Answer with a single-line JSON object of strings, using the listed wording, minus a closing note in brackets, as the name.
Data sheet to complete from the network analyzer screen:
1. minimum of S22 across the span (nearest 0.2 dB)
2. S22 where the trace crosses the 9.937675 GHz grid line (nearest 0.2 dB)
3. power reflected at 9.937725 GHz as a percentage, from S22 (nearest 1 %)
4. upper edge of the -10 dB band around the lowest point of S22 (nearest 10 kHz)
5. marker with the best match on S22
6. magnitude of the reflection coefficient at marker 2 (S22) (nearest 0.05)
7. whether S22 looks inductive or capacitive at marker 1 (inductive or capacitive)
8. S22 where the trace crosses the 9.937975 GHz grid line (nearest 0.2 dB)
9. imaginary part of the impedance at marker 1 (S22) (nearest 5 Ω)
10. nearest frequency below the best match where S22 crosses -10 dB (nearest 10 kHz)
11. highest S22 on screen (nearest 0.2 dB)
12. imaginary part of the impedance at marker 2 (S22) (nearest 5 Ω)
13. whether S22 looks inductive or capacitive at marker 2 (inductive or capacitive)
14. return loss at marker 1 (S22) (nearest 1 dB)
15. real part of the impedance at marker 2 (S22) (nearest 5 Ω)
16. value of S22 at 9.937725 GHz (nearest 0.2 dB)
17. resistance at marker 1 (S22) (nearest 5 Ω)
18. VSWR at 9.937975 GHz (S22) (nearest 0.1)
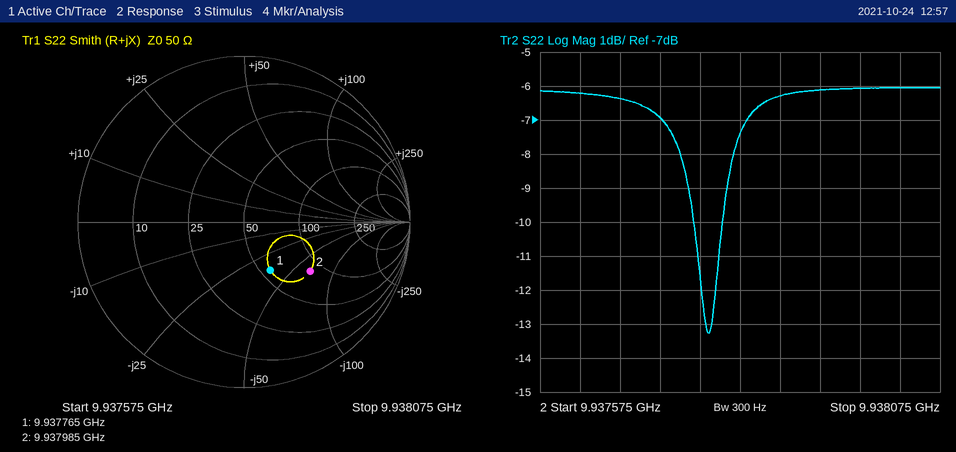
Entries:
{"minimum of S22 across the span": "-13.2 dB", "S22 where the trace crosses the 9.937675 GHz grid line": "-6.4 dB", "power reflected at 9.937725 GHz as a percentage, from S22": "20 %", "upper edge of the -10 dB band around the lowest point of S22": "9.93780 GHz", "marker with the best match on S22": "marker 1", "magnitude of the reflection coefficient at marker 2 (S22)": "0.50", "whether S22 looks inductive or capacitive at marker 1": "capacitive", "S22 where the trace crosses the 9.937975 GHz grid line": "-6.0 dB", "imaginary part of the impedance at marker 1 (S22)": "-35 Ω", "nearest frequency below the best match where S22 crosses -10 dB": "9.93777 GHz", "highest S22 on screen": "-6.0 dB", "imaginary part of the impedance at marker 2 (S22)": "-65 Ω", "whether S22 looks inductive or capacitive at marker 2": "capacitive", "return loss at marker 1 (S22)": "10 dB", "real part of the impedance at marker 2 (S22)": "85 Ω", "value of S22 at 9.937725 GHz": "-7.0 dB", "resistance at marker 1 (S22)": "55 Ω", "VSWR at 9.937975 GHz (S22)": "3.0"}
